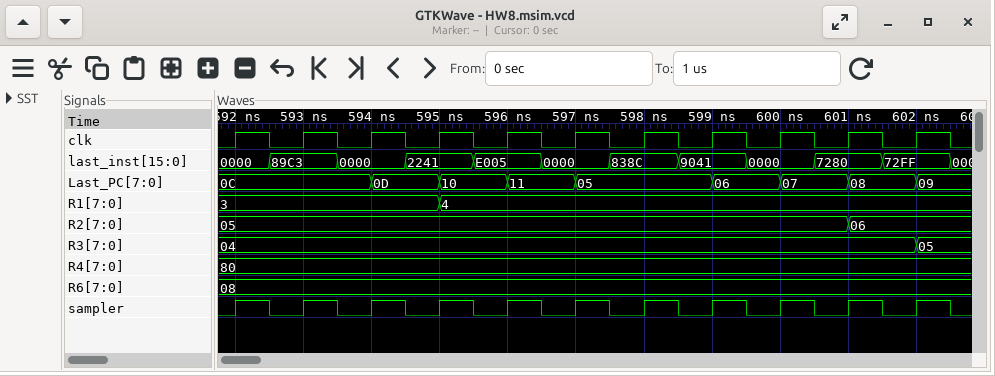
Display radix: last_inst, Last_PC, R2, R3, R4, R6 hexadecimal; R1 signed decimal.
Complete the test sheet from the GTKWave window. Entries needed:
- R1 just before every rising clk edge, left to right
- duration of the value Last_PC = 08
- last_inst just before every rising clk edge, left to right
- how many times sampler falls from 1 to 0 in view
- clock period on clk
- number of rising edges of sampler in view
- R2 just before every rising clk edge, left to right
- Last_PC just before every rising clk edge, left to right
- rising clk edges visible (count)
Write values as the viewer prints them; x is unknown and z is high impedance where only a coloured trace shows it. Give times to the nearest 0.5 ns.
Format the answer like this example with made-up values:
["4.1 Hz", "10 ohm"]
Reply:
["3, 3, 3, 3, 4, 4, 4, 4, 4, 4, 4", "1 ns", "0000, 89C3, 0000, 2241, E005, 0000, 838C, 9041, 0000, 7280, 72FF", "11", "1 ns", "11", "05, 05, 05, 05, 05, 05, 05, 05, 05, 05, 06", "0C, 0C, 0C, 0D, 10, 11, 05, 05, 06, 07, 08", "11"]
